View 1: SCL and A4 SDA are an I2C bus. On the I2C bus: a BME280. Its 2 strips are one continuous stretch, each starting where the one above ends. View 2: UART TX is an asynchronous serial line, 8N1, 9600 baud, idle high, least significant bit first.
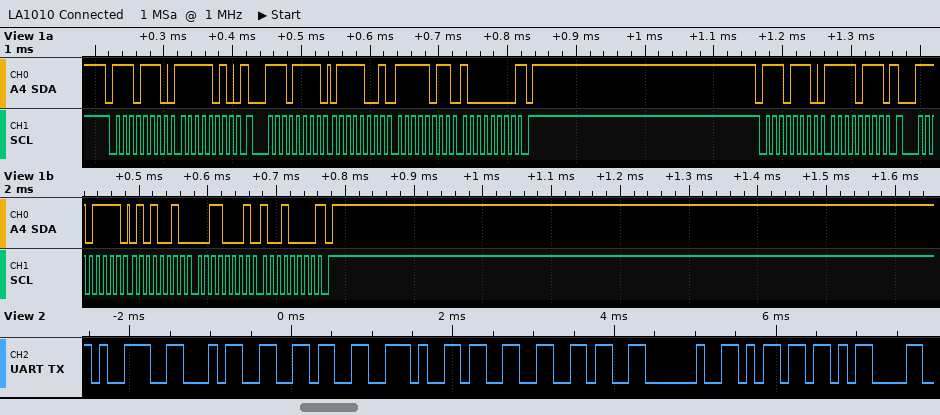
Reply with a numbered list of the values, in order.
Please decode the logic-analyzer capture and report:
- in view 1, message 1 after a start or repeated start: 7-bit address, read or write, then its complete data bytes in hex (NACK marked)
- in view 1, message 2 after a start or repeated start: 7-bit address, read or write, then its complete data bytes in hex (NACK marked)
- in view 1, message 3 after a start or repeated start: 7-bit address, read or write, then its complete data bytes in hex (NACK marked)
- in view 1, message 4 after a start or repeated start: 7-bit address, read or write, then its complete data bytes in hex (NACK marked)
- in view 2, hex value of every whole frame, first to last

1. 0x77 write: FA
2. 0x77 read: 79 FB 80 NACK
3. 0x77 write: F7
4. 0x77 read: 52 31 90 NACK
5. 39 34 36 2E 33 36 20 6D 0D
